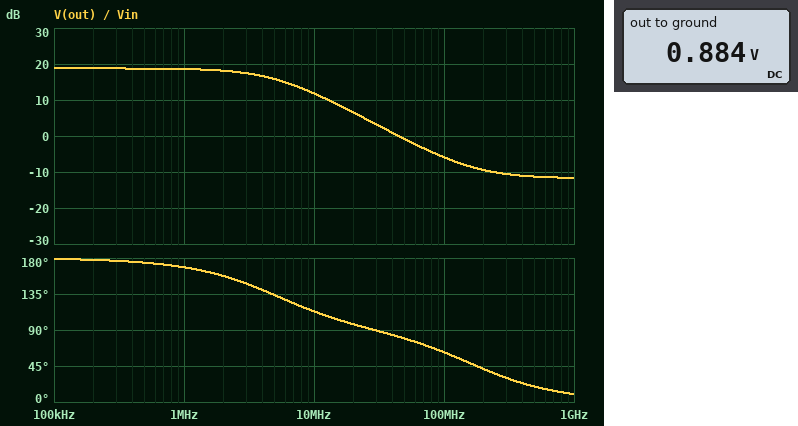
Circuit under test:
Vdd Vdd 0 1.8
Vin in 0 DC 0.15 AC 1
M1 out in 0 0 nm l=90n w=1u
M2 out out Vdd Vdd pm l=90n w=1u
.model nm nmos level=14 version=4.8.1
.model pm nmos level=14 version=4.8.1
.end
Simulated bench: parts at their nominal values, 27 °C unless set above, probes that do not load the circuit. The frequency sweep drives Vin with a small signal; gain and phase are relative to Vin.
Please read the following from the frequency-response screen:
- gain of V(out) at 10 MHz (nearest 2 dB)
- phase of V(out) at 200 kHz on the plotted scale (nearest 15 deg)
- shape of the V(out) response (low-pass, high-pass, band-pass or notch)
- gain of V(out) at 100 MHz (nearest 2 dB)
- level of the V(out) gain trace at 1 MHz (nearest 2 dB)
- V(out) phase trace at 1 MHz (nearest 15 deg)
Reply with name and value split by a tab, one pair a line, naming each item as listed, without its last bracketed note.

gain of V(out) at 10 MHz	12 dB
phase of V(out) at 200 kHz on the plotted scale	180 deg
shape of the V(out) response	low-pass
gain of V(out) at 100 MHz	-6 dB
level of the V(out) gain trace at 1 MHz	18 dB
V(out) phase trace at 1 MHz	165 deg
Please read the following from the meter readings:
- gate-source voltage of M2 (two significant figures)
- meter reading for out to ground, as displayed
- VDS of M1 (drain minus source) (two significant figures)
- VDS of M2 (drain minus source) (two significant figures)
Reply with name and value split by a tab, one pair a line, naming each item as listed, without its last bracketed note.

gate-source voltage of M2	-920 mV
meter reading for out to ground, as displayed	0.884 V
VDS of M1 (drain minus source)	880 mV
VDS of M2 (drain minus source)	-920 mV
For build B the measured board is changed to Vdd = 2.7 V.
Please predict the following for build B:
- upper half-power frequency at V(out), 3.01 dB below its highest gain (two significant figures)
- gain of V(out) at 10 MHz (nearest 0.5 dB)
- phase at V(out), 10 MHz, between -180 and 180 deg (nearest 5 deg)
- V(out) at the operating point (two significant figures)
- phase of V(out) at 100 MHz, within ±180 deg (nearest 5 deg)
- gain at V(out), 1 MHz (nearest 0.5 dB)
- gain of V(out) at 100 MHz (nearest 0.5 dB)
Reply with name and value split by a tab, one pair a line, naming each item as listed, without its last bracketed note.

upper half-power frequency at V(out), 3.01 dB below its highest gain	5.5 MHz
gain of V(out) at 10 MHz	17.0 dB
phase at V(out), 10 MHz, between -180 and 180 deg	115 deg
V(out) at the operating point	1.3 V
phase of V(out) at 100 MHz, within ±180 deg	75 deg
gain at V(out), 1 MHz	23.0 dB
gain of V(out) at 100 MHz	-1.5 dB
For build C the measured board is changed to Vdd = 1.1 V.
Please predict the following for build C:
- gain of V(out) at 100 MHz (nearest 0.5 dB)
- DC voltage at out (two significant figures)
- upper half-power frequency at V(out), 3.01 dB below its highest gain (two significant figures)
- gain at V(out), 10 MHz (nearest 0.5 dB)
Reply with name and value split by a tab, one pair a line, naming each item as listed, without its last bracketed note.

gain of V(out) at 100 MHz	-11.5 dB
DC voltage at out	350 mV
upper half-power frequency at V(out), 3.01 dB below its highest gain	6.7 MHz
gain at V(out), 10 MHz	1.0 dB
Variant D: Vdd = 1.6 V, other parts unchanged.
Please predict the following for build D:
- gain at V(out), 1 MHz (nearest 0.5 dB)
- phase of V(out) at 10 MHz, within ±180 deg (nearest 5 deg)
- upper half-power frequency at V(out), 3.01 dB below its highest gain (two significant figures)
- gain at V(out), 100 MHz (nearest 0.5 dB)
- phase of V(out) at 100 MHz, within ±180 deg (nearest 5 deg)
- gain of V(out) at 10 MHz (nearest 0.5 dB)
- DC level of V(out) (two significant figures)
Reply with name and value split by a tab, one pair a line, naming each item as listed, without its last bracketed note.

gain at V(out), 1 MHz	14.5 dB
phase of V(out) at 10 MHz, within ±180 deg	120 deg
upper half-power frequency at V(out), 3.01 dB below its highest gain	6.4 MHz
gain at V(out), 100 MHz	-7.5 dB
phase of V(out) at 100 MHz, within ±180 deg	55 deg
gain of V(out) at 10 MHz	9.5 dB
DC level of V(out)	760 mV
